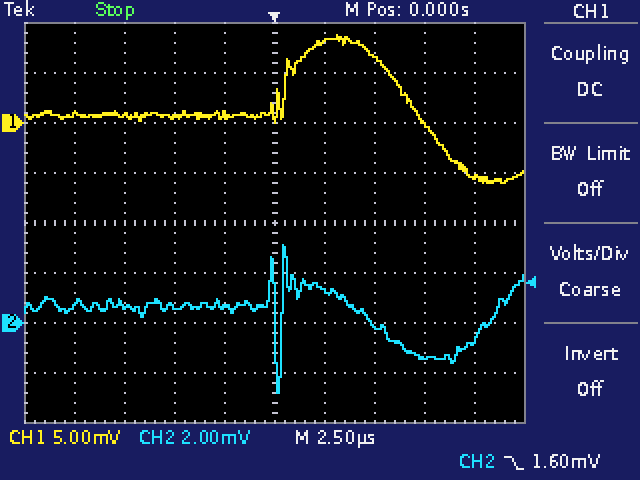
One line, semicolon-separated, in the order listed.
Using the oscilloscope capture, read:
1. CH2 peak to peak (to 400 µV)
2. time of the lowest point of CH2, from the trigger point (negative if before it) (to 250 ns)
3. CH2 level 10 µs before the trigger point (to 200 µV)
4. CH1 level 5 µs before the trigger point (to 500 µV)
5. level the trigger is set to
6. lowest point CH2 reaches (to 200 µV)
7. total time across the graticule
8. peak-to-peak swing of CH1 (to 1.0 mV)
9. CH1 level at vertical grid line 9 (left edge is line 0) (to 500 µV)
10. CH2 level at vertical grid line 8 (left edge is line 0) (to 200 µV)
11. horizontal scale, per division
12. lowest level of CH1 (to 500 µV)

6.0 mV; +250 ns; 800 µV; 500 µV; 1.60 mV; -2.8 mV; 25 µs; 15.0 mV; -5.5 mV; -1.4 mV; 2.5 µs; -6.0 mV
